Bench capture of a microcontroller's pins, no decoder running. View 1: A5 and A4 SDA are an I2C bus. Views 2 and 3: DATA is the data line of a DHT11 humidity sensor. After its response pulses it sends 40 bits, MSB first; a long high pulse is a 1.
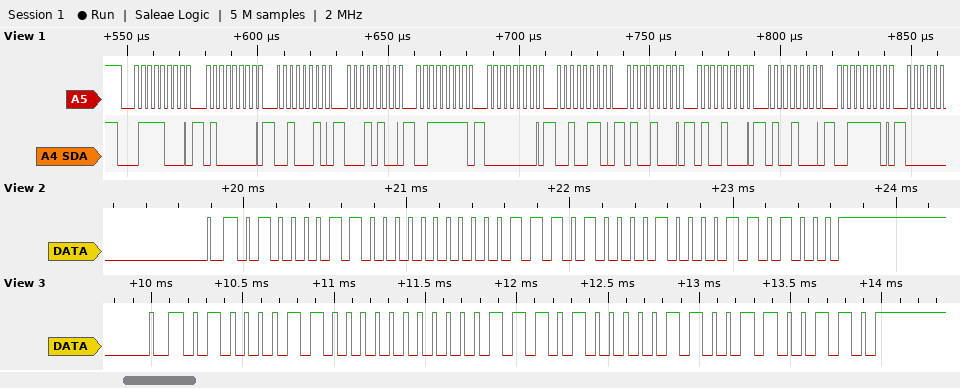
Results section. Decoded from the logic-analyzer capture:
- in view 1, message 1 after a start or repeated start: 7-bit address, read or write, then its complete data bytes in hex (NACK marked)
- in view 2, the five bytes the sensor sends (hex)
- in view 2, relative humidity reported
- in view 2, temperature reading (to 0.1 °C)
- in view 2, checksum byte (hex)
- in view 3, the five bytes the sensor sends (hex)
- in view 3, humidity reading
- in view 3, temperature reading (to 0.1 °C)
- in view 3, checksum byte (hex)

0x3C write: 40 22 14 3F 00 26 48 48 48 3E
43 00 1D 08 68
67 %
29.8 °C
0x68
43 00 1D 06 66
67 %
29.6 °C
0x66
